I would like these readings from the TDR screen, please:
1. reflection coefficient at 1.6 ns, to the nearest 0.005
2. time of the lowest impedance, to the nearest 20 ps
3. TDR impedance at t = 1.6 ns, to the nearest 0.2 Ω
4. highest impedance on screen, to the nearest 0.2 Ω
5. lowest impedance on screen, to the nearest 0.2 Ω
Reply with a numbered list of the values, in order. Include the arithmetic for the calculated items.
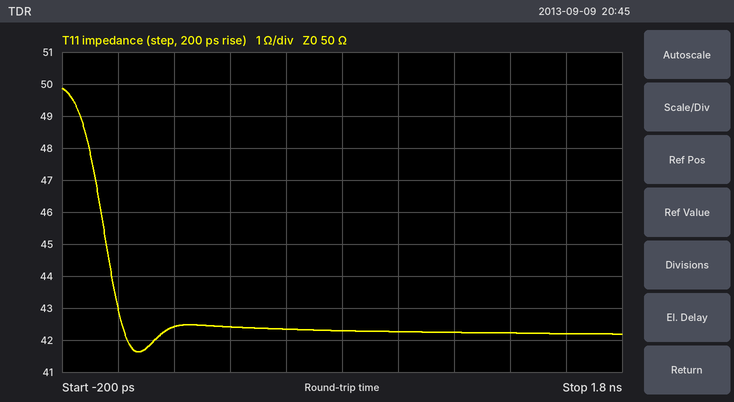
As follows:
1. (42.2 − 50)/(42.2 + 50) ≈ -0.085
2. 80 ps
3. 42.2 Ω
4. 49.8 Ω
5. 41.6 Ω
